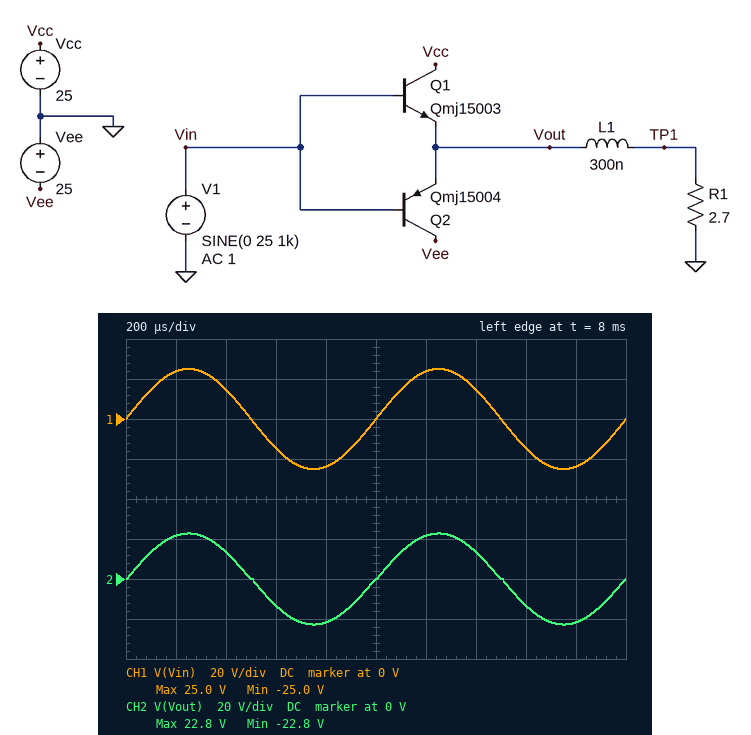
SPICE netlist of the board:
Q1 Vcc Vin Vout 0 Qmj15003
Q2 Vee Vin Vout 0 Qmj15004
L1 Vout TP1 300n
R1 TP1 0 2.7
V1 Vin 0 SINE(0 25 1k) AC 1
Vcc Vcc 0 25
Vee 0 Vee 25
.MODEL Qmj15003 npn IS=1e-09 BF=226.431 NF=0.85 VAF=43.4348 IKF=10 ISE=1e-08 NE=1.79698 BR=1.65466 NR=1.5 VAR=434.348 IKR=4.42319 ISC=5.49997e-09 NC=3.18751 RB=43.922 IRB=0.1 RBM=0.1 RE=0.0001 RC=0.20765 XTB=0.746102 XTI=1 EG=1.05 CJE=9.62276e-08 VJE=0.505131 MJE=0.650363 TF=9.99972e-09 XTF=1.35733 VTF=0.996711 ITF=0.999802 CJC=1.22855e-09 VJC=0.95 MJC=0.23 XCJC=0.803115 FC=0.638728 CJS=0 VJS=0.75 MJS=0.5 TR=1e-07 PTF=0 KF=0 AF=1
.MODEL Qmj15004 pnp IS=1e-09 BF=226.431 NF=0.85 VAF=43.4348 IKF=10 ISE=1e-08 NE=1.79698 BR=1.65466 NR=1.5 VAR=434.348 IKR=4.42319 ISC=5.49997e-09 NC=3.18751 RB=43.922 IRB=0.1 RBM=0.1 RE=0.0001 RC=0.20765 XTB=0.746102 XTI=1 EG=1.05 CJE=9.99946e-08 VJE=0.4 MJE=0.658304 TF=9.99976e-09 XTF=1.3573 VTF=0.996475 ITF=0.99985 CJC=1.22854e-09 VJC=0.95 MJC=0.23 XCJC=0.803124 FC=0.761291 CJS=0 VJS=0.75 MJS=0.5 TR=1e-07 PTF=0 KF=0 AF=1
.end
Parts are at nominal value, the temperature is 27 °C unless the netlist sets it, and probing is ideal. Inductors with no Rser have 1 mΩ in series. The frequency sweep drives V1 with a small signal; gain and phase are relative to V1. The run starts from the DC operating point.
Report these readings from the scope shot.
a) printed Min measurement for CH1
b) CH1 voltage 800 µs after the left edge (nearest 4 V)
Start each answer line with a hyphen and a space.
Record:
- -25.0 V
- -24 V
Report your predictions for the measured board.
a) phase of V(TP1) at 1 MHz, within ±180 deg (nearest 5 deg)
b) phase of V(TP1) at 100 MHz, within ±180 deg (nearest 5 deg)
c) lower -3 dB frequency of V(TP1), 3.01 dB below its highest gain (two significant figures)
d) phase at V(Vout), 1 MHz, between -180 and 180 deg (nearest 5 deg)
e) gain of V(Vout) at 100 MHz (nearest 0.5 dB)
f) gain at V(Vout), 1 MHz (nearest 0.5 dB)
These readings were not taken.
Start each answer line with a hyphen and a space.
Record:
- -5 deg
- -170 deg
- 57 kHz
- 30 deg
- -24.0 dB
- -17.5 dB
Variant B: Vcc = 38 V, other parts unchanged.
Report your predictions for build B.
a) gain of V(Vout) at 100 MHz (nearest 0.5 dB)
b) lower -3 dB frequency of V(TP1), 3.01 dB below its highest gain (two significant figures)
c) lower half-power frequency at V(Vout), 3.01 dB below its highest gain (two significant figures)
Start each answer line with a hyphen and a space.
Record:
- -23.5 dB
- 55 kHz
- 6.5 MHz
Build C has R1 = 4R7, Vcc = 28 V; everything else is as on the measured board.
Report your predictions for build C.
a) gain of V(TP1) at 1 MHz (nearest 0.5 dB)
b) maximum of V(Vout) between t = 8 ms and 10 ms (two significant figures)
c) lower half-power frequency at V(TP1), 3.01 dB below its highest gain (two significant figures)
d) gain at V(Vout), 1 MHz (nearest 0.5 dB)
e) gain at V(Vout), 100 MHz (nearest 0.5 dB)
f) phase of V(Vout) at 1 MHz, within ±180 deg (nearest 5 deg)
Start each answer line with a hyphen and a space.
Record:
- -15.0 dB
- 24 V
- 44 kHz
- -14.5 dB
- -23.5 dB
- 20 deg
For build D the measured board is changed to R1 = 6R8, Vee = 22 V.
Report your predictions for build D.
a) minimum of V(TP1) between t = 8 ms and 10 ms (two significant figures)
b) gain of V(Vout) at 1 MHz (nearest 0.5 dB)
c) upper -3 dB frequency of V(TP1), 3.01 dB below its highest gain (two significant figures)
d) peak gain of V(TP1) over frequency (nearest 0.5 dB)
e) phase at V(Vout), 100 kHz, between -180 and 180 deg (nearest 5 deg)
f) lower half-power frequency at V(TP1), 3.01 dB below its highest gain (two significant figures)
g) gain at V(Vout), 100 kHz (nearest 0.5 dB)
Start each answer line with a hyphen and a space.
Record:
- -22 V
- -12.0 dB
- 13 MHz
- -11.5 dB
- 15 deg
- 37 kHz
- -13.0 dB
